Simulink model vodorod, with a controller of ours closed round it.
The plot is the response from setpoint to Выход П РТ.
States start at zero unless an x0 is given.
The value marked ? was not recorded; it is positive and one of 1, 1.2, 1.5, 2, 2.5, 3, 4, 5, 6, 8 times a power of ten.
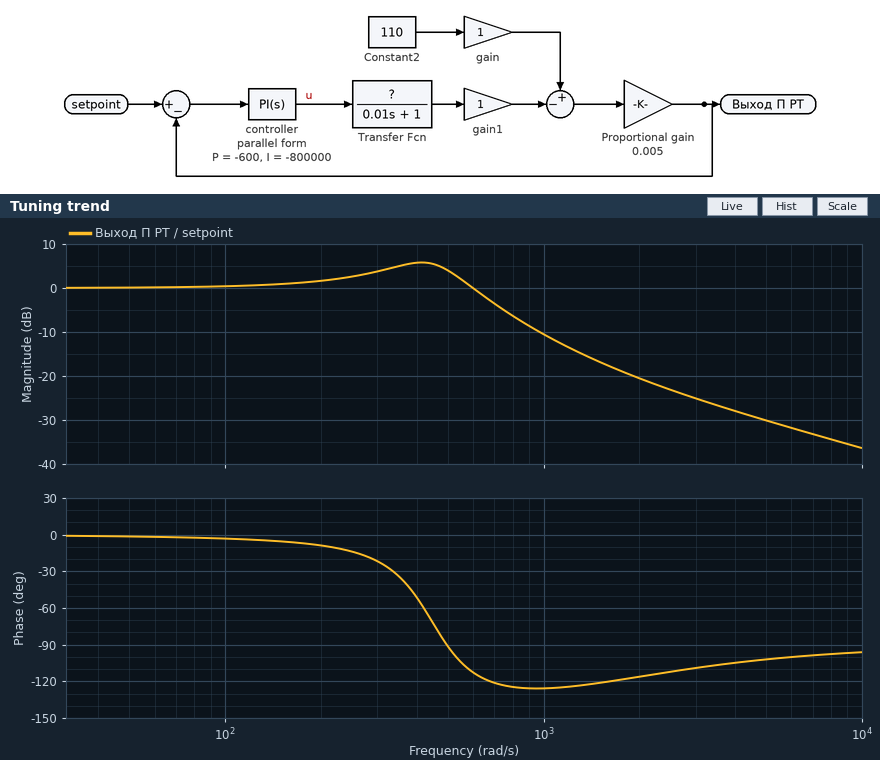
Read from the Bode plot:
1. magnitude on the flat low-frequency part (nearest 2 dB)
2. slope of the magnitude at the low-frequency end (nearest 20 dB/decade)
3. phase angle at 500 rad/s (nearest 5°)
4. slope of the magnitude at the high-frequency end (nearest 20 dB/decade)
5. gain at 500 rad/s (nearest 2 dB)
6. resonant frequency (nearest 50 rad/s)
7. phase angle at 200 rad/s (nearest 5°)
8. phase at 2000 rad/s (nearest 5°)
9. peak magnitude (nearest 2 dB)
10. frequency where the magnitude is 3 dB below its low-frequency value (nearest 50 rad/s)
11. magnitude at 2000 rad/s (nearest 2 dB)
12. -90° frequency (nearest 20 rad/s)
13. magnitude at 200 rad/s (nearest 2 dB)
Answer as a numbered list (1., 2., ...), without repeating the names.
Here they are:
1. 0 dB
2. 0 dB/decade
3. -90°
4. -20 dB/decade
5. 4 dB
6. 400 rad/s
7. -10°
8. -115°
9. 6 dB
10. 700 rad/s
11. -20 dB
12. 500 rad/s
13. 2 dB
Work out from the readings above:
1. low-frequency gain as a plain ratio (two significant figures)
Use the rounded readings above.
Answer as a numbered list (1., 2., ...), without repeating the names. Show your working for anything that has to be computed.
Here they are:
1. 10^(0 / 20) = 1.0
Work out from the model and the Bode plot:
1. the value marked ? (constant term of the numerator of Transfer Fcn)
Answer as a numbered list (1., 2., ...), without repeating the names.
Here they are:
1. 0.5
